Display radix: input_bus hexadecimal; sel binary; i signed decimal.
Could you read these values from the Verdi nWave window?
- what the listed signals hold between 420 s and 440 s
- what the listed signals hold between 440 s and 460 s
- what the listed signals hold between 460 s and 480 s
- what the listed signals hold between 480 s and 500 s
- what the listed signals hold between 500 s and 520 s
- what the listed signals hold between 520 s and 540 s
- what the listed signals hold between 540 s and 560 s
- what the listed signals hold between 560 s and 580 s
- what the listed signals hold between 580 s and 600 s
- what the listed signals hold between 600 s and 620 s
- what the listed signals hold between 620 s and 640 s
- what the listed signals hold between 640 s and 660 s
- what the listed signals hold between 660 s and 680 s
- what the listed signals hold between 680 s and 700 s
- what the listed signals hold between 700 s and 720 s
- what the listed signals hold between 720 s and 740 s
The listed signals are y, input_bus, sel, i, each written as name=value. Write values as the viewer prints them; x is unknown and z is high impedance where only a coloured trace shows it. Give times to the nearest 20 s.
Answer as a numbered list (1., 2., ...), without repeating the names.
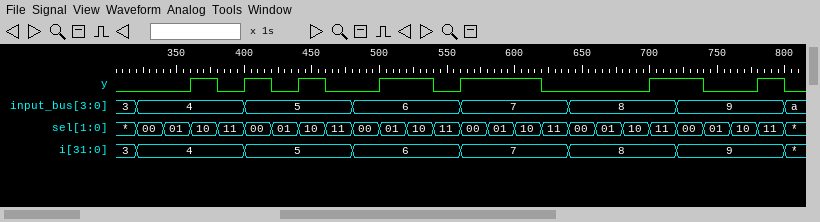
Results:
1. y=0, input_bus=5, sel=01, i=5
2. y=1, input_bus=5, sel=10, i=5
3. y=0, input_bus=5, sel=11, i=5
4. y=0, input_bus=6, sel=00, i=6
5. y=1, input_bus=6, sel=01, i=6
6. y=1, input_bus=6, sel=10, i=6
7. y=0, input_bus=6, sel=11, i=6
8. y=1, input_bus=7, sel=00, i=7
9. y=1, input_bus=7, sel=01, i=7
10. y=1, input_bus=7, sel=10, i=7
11. y=0, input_bus=7, sel=11, i=7
12. y=0, input_bus=8, sel=00, i=8
13. y=0, input_bus=8, sel=01, i=8
14. y=0, input_bus=8, sel=10, i=8
15. y=1, input_bus=8, sel=11, i=8
16. y=1, input_bus=9, sel=00, i=9
